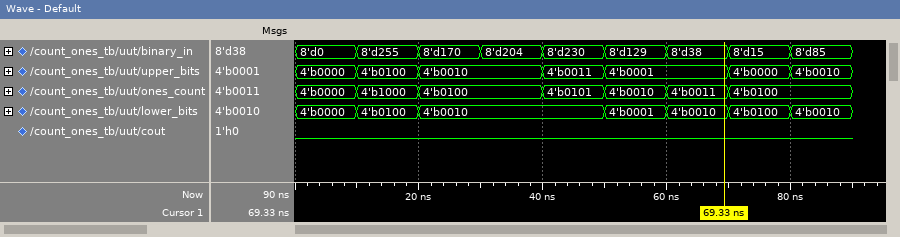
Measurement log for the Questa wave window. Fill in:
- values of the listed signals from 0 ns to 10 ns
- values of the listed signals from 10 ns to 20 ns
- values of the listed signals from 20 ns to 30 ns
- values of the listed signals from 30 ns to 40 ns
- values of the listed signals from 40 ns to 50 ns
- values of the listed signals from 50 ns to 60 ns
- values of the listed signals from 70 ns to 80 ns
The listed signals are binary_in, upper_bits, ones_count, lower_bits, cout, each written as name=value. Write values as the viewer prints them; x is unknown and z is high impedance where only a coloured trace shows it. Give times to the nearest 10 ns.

binary_in=8'd0, upper_bits=4'b0000, ones_count=4'b0000, lower_bits=4'b0000, cout=0
binary_in=8'd255, upper_bits=4'b0100, ones_count=4'b1000, lower_bits=4'b0100, cout=0
binary_in=8'd170, upper_bits=4'b0010, ones_count=4'b0100, lower_bits=4'b0010, cout=0
binary_in=8'd204, upper_bits=4'b0010, ones_count=4'b0100, lower_bits=4'b0010, cout=0
binary_in=8'd230, upper_bits=4'b0011, ones_count=4'b0101, lower_bits=4'b0010, cout=0
binary_in=8'd129, upper_bits=4'b0001, ones_count=4'b0010, lower_bits=4'b0001, cout=0
binary_in=8'd15, upper_bits=4'b0000, ones_count=4'b0100, lower_bits=4'b0100, cout=0
